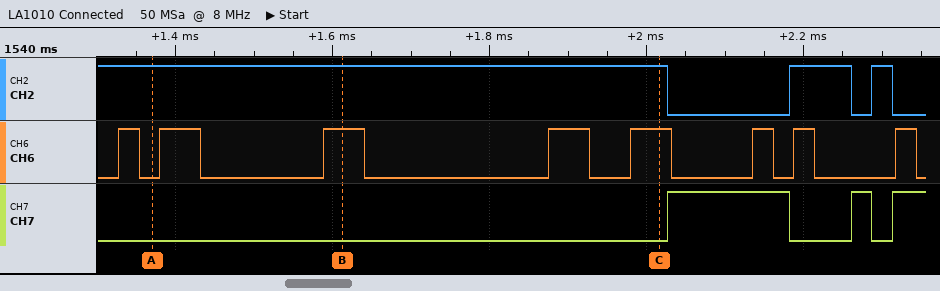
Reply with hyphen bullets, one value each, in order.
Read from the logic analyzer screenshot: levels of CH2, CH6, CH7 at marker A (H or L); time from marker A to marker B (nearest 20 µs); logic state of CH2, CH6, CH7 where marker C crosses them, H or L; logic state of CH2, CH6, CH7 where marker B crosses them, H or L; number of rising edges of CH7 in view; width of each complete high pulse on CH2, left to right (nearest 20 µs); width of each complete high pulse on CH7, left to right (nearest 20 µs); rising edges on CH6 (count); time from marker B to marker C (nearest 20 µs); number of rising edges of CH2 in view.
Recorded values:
- CH2=H, CH6=L, CH7=L
- 240 µs
- CH2=H, CH6=H, CH7=L
- CH2=H, CH6=H, CH7=L
- 3
- 80 µs, 20 µs
- 160 µs, 20 µs
- 8
- 400 µs
- 2
